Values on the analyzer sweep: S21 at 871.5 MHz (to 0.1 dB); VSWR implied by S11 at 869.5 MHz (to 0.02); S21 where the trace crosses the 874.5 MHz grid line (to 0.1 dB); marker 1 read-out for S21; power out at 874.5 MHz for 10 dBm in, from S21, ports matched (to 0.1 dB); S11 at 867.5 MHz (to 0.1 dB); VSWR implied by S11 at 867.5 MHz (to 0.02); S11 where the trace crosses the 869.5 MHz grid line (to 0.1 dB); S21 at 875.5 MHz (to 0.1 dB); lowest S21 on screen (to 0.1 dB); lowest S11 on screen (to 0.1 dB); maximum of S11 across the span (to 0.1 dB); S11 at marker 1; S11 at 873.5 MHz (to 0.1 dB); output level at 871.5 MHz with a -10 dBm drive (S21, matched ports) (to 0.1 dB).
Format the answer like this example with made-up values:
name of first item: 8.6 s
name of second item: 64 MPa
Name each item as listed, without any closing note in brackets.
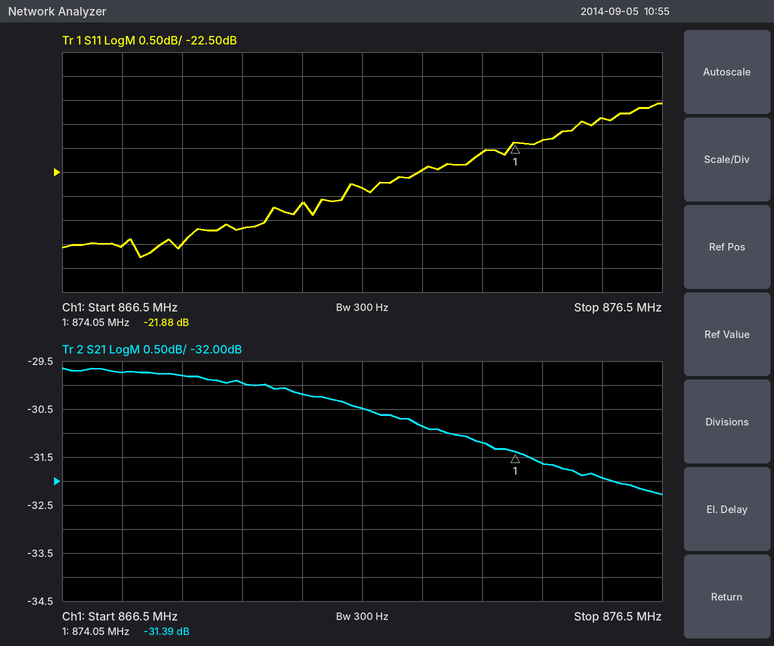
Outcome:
S21 at 871.5 MHz: -30.5 dB
VSWR implied by S11 at 869.5 MHz: 1.14
S21 where the trace crosses the 874.5 MHz grid line: -31.6 dB
marker 1 read-out for S21: -31.39 dB
power out at 874.5 MHz for 10 dBm in, from S21, ports matched: -21.6 dBm
S11 at 867.5 MHz: -24.0 dB
VSWR implied by S11 at 867.5 MHz: 1.14
S11 where the trace crosses the 869.5 MHz grid line: -23.7 dB
S21 at 875.5 MHz: -31.9 dB
lowest S21 on screen: -32.3 dB
lowest S11 on screen: -24.3 dB
maximum of S11 across the span: -21.1 dB
S11 at marker 1: -21.88 dB
S11 at 873.5 MHz: -22.1 dB
output level at 871.5 MHz with a -10 dBm drive (S21, matched ports): -40.5 dBm
